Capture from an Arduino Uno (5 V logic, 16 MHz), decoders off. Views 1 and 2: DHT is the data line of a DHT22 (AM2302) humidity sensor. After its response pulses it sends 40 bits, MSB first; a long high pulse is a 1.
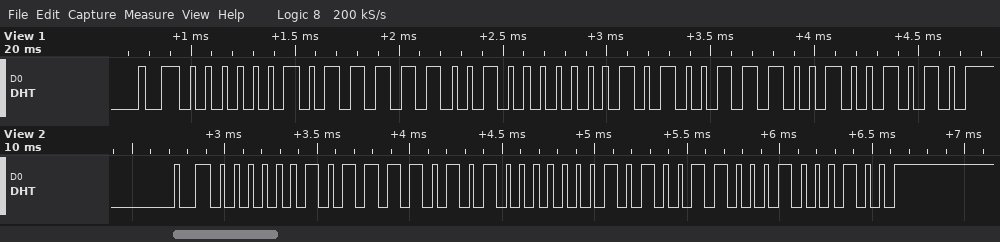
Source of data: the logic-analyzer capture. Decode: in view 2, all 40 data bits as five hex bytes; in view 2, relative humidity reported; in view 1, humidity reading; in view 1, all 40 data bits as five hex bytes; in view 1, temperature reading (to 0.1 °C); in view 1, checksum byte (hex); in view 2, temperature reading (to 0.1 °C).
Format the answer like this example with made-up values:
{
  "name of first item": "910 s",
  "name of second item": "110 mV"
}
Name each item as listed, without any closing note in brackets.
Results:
{
  "in view 2, all 40 data bits as five hex bytes": "02 F5 01 4C 44",
  "in view 2, relative humidity reported": "75.7 %",
  "in view 1, humidity reading": "76.1 %",
  "in view 1, all 40 data bits as five hex bytes": "02 F9 01 4E 4A",
  "in view 1, temperature reading": "33.4 °C",
  "in view 1, checksum byte": "0x4A",
  "in view 2, temperature reading": "33.2 °C"
}
